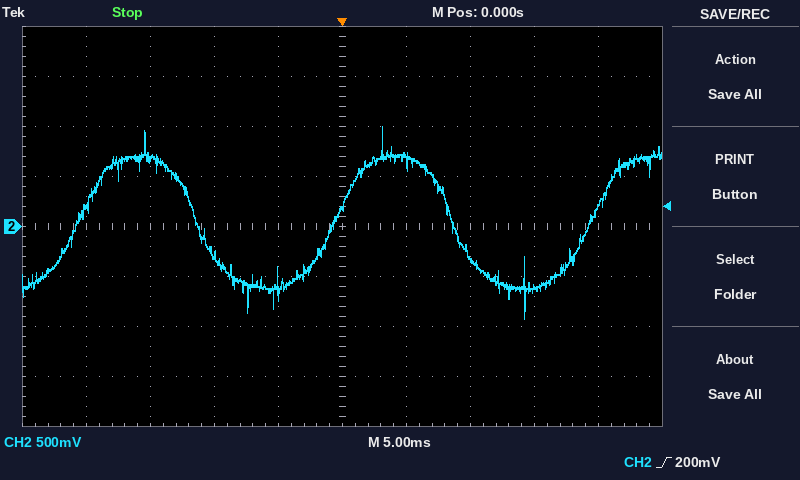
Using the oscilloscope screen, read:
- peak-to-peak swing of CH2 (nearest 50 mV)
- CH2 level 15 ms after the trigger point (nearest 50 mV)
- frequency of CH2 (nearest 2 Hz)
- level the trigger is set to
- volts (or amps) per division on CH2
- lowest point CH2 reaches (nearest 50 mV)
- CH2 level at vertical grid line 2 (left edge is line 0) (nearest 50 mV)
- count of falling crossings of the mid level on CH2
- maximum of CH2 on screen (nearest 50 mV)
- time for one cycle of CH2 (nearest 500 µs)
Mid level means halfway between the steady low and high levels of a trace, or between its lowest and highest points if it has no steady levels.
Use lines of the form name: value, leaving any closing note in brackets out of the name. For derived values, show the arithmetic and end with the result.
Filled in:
peak-to-peak swing of CH2: 1.00 V − (-900 mV) = 1.90 V
CH2 level 15 ms after the trigger point: -600 mV
frequency of CH2: 1 / 20.0 ms ≈ 50 Hz
level the trigger is set to: 200 mV
volts (or amps) per division on CH2: 500 mV
lowest point CH2 reaches: -900 mV
CH2 level at vertical grid line 2 (left edge is line 0): 700 mV
count of falling crossings of the mid level on CH2: 2
maximum of CH2 on screen: 1.00 V
time for one cycle of CH2: 20.0 ms
